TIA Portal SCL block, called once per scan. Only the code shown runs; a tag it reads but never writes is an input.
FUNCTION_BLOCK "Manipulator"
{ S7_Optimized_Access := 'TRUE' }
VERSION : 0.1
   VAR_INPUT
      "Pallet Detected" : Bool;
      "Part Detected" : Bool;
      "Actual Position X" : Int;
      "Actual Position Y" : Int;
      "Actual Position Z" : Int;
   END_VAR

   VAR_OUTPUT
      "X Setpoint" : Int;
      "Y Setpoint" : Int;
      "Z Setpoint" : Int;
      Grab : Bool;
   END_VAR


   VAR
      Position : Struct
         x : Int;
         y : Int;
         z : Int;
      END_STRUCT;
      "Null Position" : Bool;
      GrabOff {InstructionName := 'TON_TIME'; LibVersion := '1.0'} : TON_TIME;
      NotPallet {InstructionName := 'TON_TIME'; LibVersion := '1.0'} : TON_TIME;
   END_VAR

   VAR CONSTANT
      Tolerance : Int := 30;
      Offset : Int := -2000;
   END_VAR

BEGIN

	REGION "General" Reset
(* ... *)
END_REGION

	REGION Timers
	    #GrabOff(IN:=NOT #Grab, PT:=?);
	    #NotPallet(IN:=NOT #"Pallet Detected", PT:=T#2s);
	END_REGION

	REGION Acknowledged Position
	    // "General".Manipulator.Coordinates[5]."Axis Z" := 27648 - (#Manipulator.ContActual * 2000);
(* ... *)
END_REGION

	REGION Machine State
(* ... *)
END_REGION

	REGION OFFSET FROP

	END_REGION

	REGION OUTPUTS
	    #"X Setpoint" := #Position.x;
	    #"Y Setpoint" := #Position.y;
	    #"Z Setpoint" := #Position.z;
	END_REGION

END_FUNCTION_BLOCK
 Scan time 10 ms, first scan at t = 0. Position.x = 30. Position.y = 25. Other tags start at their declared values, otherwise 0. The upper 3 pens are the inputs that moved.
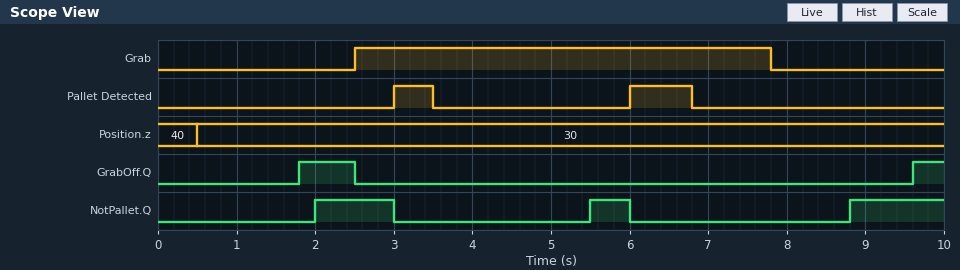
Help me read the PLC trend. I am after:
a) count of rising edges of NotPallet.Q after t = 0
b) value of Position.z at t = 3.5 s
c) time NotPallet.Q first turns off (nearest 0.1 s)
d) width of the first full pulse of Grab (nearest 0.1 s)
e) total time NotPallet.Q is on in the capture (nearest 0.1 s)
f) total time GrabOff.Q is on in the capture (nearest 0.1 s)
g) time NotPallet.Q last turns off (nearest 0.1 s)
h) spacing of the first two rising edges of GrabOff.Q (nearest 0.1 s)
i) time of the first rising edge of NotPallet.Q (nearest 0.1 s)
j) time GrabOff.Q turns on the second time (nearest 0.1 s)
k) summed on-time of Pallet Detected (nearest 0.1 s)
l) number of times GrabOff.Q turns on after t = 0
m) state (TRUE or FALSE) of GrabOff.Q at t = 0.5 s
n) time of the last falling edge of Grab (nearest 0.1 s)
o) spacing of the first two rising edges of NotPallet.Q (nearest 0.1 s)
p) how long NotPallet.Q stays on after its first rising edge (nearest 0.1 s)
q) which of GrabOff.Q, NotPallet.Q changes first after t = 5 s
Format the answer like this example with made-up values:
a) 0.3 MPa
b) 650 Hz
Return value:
a) 3
b) 30
c) 3.0 s
d) 5.3 s
e) 2.7 s
f) 1.1 s
g) 6.0 s
h) 7.8 s
i) 2.0 s
j) 9.6 s
k) 1.3 s
l) 2
m) FALSE
n) 7.8 s
o) 3.5 s
p) 1.0 s
q) NotPallet.Q
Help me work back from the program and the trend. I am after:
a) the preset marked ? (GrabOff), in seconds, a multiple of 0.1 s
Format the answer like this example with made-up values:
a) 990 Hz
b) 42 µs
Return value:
a) 1.8 s
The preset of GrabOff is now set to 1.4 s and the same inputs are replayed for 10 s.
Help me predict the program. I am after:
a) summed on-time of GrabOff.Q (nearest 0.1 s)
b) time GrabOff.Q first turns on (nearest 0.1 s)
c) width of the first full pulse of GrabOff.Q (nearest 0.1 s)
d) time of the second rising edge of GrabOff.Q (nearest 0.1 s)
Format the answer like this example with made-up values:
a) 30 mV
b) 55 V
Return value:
a) 1.9 s
b) 1.4 s
c) 1.1 s
d) 9.2 s
